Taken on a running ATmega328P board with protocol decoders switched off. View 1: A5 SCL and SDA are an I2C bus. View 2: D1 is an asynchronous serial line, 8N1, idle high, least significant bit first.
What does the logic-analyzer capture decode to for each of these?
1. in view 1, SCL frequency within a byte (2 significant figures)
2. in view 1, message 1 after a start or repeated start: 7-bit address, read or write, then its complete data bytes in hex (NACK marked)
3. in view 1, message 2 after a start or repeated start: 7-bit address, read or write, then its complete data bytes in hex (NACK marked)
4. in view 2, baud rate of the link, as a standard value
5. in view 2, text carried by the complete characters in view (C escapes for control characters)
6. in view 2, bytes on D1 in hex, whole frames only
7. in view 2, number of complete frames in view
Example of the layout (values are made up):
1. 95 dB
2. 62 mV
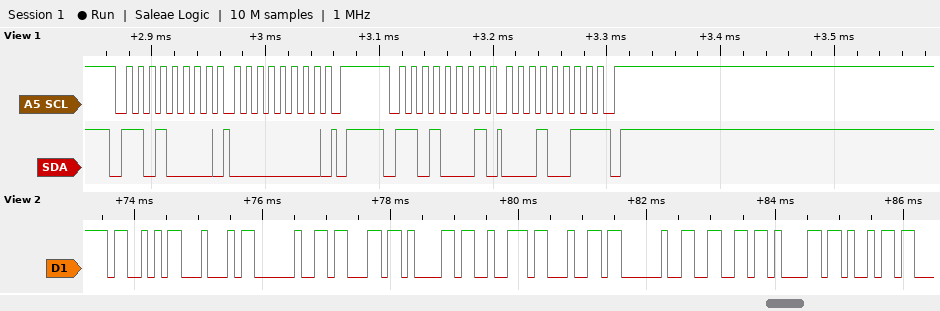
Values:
1. 100 kHz
2. 0x68 write: 00
3. 0x68 read: 13 NACK
4. 9600 baud
5. "SD card fai"
6. 53 44 20 63 61 72 64 20 66 61 69
7. 11
